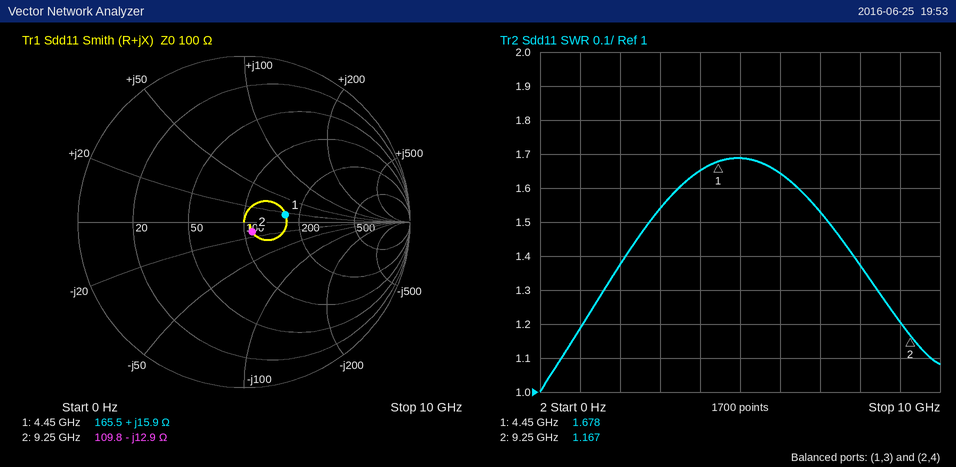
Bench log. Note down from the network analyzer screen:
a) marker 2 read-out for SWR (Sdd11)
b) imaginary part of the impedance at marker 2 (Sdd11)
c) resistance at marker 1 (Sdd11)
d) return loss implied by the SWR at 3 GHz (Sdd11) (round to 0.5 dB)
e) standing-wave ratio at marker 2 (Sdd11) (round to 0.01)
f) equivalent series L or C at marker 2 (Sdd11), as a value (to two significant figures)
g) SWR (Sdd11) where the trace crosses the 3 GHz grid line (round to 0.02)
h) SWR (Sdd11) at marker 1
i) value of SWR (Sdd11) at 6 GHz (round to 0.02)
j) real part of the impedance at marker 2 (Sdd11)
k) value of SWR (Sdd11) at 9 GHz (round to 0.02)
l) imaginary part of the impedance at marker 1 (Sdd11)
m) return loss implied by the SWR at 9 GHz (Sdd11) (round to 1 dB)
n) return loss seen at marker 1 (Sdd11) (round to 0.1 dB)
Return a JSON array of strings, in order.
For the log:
["1.167", "-12.9 Ω", "165.5 Ω", "13.5 dB", "1.17", "1.3 pF", "1.54", "1.678", "1.64", "109.8 Ω", "1.20", "+15.9 Ω", "21 dB", "11.9 dB"]
